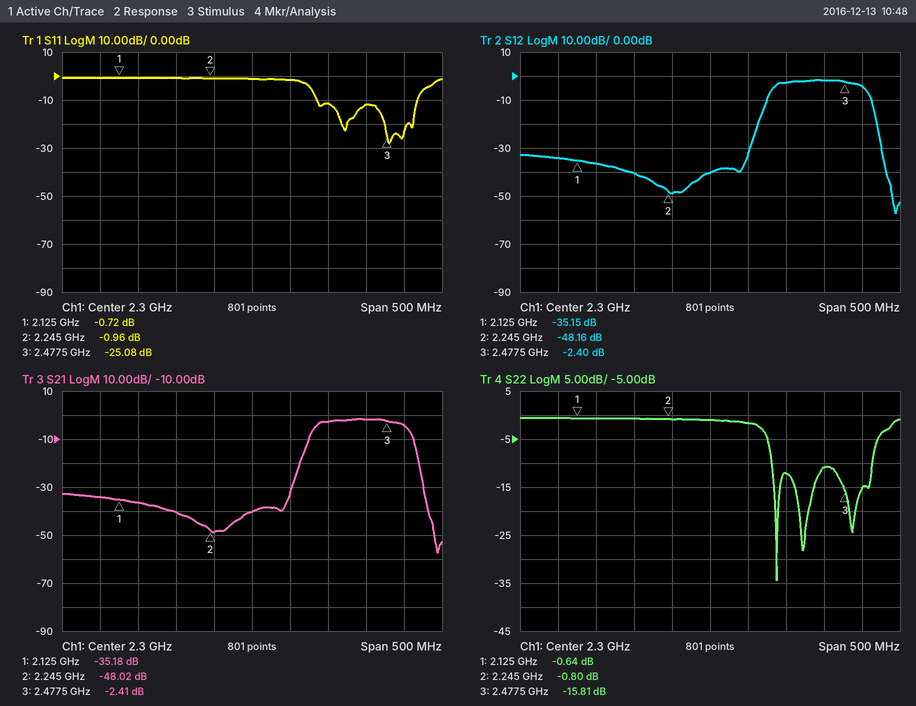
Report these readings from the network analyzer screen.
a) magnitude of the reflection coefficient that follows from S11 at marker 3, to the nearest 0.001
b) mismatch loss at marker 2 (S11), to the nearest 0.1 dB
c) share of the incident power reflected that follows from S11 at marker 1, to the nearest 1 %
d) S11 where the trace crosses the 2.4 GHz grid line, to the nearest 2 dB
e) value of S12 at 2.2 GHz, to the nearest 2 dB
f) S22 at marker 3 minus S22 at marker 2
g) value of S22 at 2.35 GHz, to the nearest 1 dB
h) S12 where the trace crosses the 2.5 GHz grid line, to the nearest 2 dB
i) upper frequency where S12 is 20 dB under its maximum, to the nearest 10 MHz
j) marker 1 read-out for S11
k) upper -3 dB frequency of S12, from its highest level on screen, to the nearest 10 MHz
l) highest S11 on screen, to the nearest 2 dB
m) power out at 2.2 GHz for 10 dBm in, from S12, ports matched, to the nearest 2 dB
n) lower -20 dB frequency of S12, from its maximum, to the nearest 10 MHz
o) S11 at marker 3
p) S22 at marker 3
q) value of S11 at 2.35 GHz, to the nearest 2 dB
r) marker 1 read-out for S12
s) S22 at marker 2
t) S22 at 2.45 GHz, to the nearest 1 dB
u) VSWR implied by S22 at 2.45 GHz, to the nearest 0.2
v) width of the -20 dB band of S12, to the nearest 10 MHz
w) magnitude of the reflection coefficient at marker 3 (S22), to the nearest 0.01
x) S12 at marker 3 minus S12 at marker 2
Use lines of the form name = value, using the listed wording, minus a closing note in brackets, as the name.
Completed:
magnitude of the reflection coefficient that follows from S11 at marker 3, to the nearest 0.001 = 0.056
mismatch loss at marker 2 (S11), to the nearest 0.1 dB = 7.0 dB
share of the incident power reflected that follows from S11 at marker 1, to the nearest 1 % = 85 %
S11 where the trace crosses the 2.4 GHz grid line, to the nearest 2 dB = -12 dB
value of S12 at 2.2 GHz, to the nearest 2 dB = -40 dB
S22 at marker 3 minus S22 at marker 2 = -15.01 dB
value of S22 at 2.35 GHz, to the nearest 1 dB = -2 dB
S12 where the trace crosses the 2.5 GHz grid line, to the nearest 2 dB = -4 dB
upper frequency where S12 is 20 dB under its maximum, to the nearest 10 MHz = 2.52 GHz
marker 1 read-out for S11 = -0.72 dB
upper -3 dB frequency of S12, from its highest level on screen, to the nearest 10 MHz = 2.50 GHz
highest S11 on screen, to the nearest 2 dB = 0 dB
power out at 2.2 GHz for 10 dBm in, from S12, ports matched, to the nearest 2 dB = -30 dBm
lower -20 dB frequency of S12, from its maximum, to the nearest 10 MHz = 2.36 GHz
S11 at marker 3 = -25.08 dB
S22 at marker 3 = -15.81 dB
value of S11 at 2.35 GHz, to the nearest 2 dB = -2 dB
marker 1 read-out for S12 = -35.15 dB
S22 at marker 2 = -0.80 dB
S22 at 2.45 GHz, to the nearest 1 dB = -11 dB
VSWR implied by S22 at 2.45 GHz, to the nearest 0.2 = 1.8
width of the -20 dB band of S12, to the nearest 10 MHz = 160 MHz
magnitude of the reflection coefficient at marker 3 (S22), to the nearest 0.01 = 0.16
S12 at marker 3 minus S12 at marker 2 = 45.76 dB
